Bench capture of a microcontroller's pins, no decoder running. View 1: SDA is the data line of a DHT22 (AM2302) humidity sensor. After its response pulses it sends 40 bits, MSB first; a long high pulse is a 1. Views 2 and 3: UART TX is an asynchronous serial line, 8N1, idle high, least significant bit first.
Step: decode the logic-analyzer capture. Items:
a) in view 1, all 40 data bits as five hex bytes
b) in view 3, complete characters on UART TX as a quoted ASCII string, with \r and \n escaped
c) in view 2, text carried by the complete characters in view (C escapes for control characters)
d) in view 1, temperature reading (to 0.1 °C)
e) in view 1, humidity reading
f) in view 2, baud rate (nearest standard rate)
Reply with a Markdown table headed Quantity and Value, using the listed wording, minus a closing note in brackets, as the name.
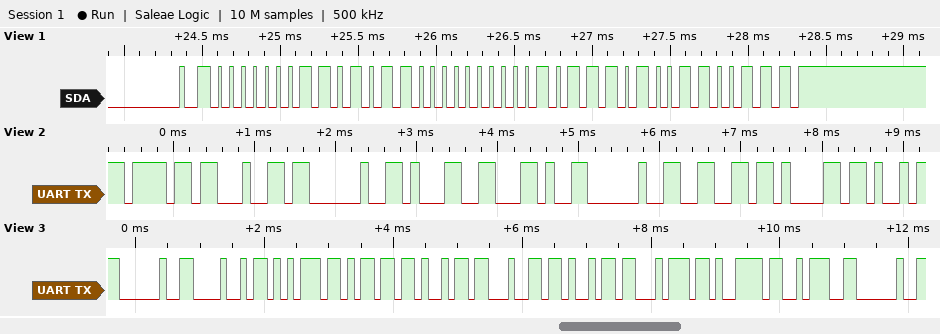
| Quantity | Value |
|---|---|
| in view 1, all 40 data bits as five hex bytes | 01 AC 00 BA 67 |
| in view 3, complete characters on UART TX as a quoted ASCII string, with \r and \n escaped | " Humidity: " |
| in view 2, text carried by the complete characters in view | "od 1, fa" |
| in view 1, temperature reading | 18.6 °C |
| in view 1, humidity reading | 42.8 % |
| in view 2, baud rate | 9600 baud |
